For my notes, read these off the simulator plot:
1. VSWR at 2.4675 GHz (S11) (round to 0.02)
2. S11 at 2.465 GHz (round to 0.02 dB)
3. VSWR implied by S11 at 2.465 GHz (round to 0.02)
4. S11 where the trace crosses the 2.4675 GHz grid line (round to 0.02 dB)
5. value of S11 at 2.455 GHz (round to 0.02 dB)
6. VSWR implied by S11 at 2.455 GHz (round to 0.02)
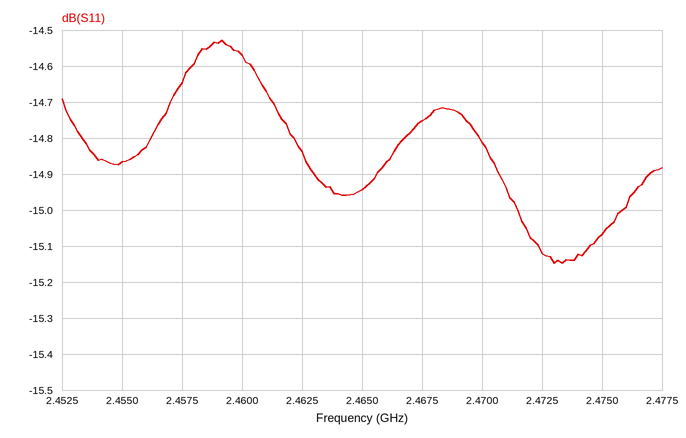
1.44
-14.94 dB
1.44
-14.76 dB
-14.86 dB
1.44
